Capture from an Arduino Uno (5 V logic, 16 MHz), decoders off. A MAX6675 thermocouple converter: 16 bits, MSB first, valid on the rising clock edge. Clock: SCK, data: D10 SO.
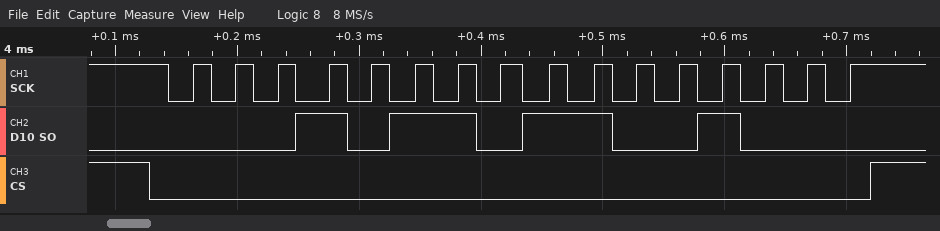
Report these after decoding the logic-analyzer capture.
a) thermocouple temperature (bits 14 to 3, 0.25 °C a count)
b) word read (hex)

182.25 °C
0x16C8
